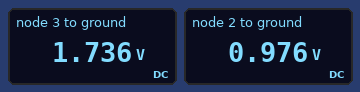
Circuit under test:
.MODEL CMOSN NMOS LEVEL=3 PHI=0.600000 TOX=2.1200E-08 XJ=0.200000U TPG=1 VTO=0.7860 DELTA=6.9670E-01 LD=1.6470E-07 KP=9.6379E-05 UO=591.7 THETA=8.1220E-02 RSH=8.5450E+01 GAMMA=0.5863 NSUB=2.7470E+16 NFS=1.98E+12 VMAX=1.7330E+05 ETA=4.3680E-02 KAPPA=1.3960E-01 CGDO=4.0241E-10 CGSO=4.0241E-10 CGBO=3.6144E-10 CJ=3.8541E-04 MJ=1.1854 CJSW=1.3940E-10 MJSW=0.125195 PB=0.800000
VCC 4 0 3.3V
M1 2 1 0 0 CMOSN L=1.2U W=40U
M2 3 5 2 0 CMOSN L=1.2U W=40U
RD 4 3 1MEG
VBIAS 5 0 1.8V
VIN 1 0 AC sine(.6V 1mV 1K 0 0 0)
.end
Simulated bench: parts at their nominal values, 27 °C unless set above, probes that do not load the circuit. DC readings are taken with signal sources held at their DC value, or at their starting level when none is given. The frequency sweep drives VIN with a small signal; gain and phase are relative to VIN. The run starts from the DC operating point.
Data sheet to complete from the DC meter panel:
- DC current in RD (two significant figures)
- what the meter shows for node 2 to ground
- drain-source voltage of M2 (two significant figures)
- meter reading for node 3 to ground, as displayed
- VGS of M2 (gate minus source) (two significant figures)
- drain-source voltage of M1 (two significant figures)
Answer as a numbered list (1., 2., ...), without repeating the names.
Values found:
1. 1.6 µA
2. 0.976 V
3. 760 mV
4. 1.736 V
5. 820 mV
6. 980 mV
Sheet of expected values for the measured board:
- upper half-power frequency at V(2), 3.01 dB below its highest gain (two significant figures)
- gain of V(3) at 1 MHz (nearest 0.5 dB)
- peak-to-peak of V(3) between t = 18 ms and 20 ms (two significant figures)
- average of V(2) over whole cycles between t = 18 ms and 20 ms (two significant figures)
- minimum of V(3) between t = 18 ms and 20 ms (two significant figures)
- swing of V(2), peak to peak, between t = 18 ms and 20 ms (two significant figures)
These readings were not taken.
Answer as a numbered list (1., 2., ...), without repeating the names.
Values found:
1. 15 MHz
2. 25.0 dB
3. 35 mV
4. 980 mV
5. 1.7 V
6. 2.5 mV
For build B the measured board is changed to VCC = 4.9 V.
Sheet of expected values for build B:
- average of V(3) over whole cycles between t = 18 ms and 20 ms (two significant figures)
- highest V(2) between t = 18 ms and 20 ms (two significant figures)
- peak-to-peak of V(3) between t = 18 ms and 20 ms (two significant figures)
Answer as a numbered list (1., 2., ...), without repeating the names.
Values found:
1. 3.3 V
2. 1.0 V
3. 36 mV
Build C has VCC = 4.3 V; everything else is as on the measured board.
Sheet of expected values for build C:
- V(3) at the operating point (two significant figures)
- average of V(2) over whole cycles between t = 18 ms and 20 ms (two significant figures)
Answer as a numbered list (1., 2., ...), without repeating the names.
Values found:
1. 2.7 V
2. 1.0 V
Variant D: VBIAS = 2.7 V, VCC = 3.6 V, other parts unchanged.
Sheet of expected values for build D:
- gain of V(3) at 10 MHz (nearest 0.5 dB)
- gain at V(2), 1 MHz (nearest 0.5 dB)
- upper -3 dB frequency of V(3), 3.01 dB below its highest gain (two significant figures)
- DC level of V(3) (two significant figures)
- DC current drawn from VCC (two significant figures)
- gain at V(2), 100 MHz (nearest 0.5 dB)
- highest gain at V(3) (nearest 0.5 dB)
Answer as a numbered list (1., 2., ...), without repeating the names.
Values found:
1. 11.0 dB
2. 21.5 dB
3. 2.8 MHz
4. 1.6 V
5. 2.0 µA
6. -8.5 dB
7. 22.5 dB
